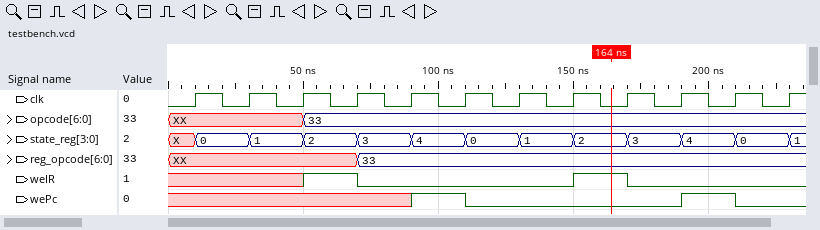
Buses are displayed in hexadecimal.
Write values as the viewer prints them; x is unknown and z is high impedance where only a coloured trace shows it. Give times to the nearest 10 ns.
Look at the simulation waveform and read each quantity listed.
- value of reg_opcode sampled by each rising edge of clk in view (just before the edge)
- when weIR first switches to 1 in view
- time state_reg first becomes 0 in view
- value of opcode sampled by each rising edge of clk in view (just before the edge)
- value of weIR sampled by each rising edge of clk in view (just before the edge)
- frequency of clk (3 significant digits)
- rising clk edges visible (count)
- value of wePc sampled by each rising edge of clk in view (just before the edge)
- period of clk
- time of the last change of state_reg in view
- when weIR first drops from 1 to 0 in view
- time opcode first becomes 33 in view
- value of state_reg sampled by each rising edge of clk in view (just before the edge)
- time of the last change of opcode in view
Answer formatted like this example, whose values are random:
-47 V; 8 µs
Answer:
XX, XX, XX, XX, 33, 33, 33, 33, 33, 33, 33, 33; 50 ns; 10 ns; XX, XX, XX, 33, 33, 33, 33, 33, 33, 33, 33, 33; x x x 1 0 0 0 0 1 0 0 0; 50.0 MHz; 12; x x x x x 1 0 0 0 0 1 0; 20 ns; 230 ns; 70 ns; 50 ns; X, 0, 1, 2, 3, 4, 0, 1, 2, 3, 4, 0; 50 ns
